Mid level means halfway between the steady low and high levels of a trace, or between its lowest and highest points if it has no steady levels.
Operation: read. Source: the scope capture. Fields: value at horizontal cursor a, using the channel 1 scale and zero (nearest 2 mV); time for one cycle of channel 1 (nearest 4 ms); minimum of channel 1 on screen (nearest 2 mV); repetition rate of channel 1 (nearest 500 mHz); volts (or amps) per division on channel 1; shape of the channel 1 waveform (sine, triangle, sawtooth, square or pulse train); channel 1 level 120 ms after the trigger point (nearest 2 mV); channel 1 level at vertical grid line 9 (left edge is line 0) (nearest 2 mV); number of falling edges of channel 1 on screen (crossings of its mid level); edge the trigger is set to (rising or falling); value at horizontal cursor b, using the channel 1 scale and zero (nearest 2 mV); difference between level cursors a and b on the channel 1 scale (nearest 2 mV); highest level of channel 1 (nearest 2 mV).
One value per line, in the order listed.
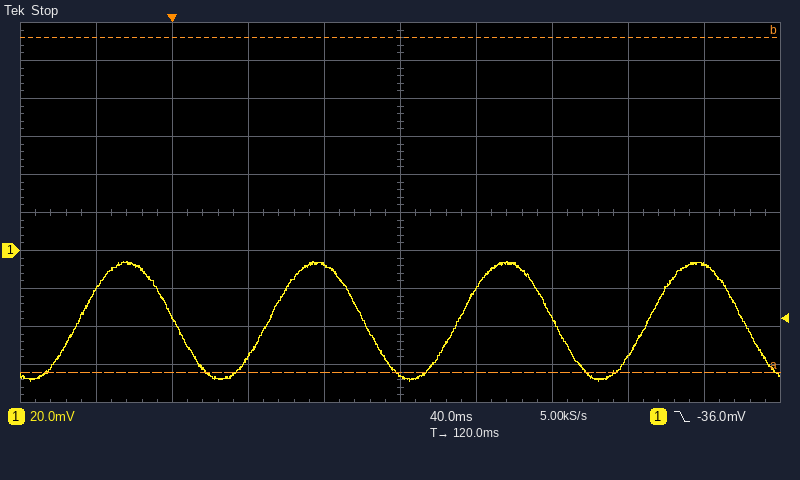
-64 mV
100 ms
-68 mV
10.0 Hz
20 mV
sine
-66 mV
-8 mV
4
falling
112 mV
176 mV
-6 mV
